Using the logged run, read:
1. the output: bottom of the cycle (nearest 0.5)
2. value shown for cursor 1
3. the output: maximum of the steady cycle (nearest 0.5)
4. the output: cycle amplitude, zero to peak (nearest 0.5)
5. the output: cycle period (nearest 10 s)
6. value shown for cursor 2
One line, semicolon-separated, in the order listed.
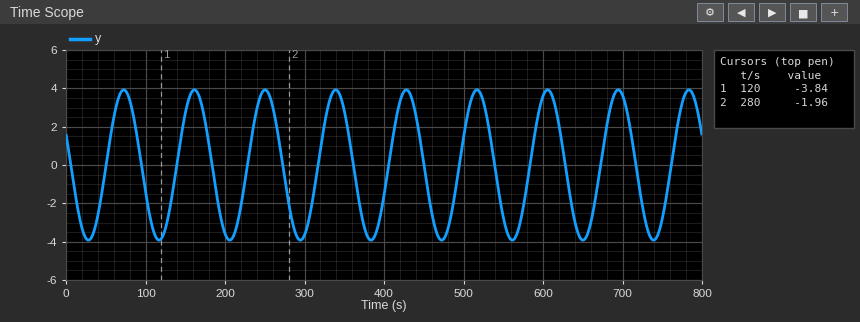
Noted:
-4.0; -3.84; 4.0; 4.0; 90 s; -1.96
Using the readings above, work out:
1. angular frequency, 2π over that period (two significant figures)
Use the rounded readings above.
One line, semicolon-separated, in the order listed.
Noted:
0.070 rad/s
